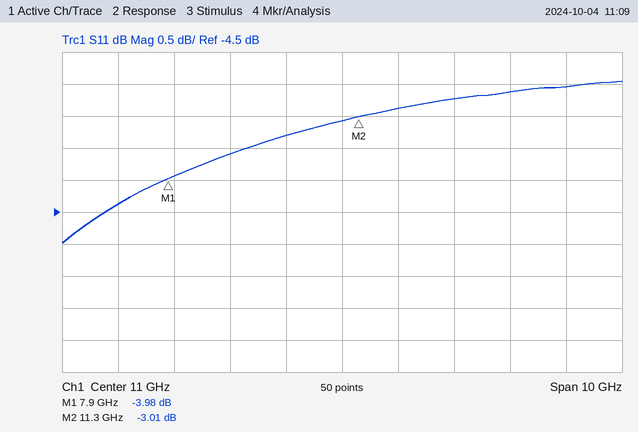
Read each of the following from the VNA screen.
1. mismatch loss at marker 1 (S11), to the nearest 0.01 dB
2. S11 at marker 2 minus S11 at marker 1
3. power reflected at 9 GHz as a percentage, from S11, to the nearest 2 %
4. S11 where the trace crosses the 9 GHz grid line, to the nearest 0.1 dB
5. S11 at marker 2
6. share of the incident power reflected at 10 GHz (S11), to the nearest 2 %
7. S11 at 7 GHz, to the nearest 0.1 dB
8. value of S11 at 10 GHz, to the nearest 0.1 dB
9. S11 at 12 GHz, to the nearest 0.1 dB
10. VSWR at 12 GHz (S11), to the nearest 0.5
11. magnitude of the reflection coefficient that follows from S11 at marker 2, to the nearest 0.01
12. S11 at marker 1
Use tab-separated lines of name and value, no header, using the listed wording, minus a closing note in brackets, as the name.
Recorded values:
mismatch loss at marker 1 (S11), to the nearest 0.01 dB	2.22 dB
S11 at marker 2 minus S11 at marker 1	0.97 dB
power reflected at 9 GHz as a percentage, from S11, to the nearest 2 %	44 %
S11 where the trace crosses the 9 GHz grid line, to the nearest 0.1 dB	-3.6 dB
S11 at marker 2	-3.01 dB
share of the incident power reflected at 10 GHz (S11), to the nearest 2 %	46 %
S11 at 7 GHz, to the nearest 0.1 dB	-4.4 dB
value of S11 at 10 GHz, to the nearest 0.1 dB	-3.3 dB
S11 at 12 GHz, to the nearest 0.1 dB	-2.9 dB
VSWR at 12 GHz (S11), to the nearest 0.5	6.0
magnitude of the reflection coefficient that follows from S11 at marker 2, to the nearest 0.01	0.71
S11 at marker 1	-3.98 dB
